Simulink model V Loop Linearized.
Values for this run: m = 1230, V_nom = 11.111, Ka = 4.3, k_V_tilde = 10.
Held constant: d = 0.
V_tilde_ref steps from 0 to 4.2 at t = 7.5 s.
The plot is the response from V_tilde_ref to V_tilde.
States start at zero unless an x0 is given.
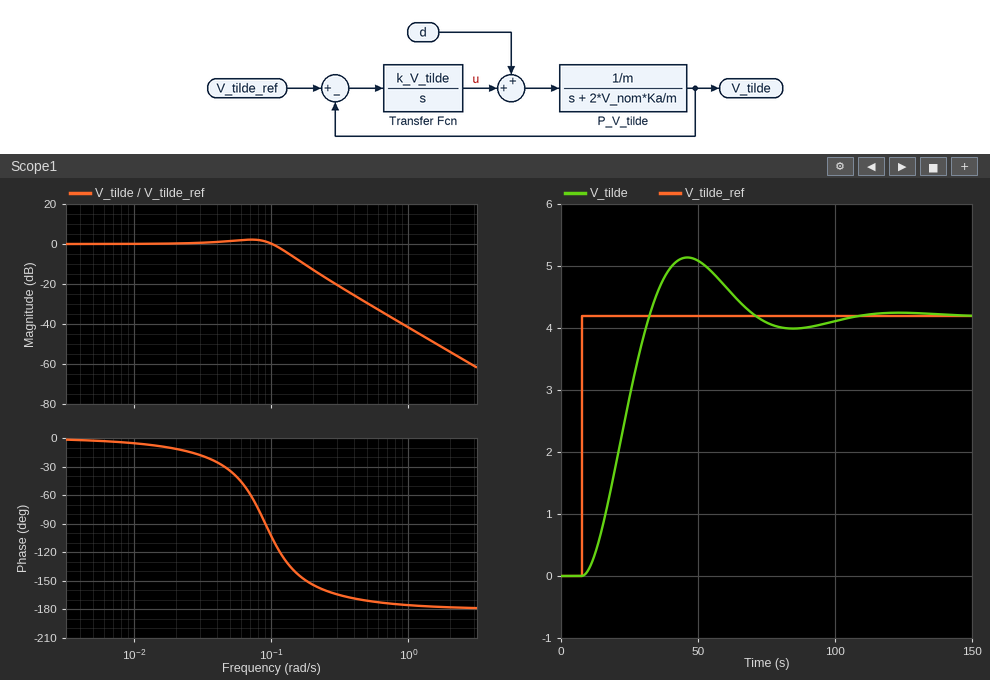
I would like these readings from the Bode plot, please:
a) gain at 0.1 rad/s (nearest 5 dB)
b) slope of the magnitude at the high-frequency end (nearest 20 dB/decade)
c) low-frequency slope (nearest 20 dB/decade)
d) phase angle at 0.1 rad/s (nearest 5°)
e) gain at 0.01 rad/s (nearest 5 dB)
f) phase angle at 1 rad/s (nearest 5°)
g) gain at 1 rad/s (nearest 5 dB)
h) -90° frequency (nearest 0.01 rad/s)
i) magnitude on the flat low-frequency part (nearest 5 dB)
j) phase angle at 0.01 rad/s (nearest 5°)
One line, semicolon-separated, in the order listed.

0 dB; -40 dB/decade; 0 dB/decade; -105°; 0 dB; -175°; -40 dB; 0.09 rad/s; 0 dB; -5°
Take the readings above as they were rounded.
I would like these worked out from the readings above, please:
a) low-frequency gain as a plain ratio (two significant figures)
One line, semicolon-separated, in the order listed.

1.0
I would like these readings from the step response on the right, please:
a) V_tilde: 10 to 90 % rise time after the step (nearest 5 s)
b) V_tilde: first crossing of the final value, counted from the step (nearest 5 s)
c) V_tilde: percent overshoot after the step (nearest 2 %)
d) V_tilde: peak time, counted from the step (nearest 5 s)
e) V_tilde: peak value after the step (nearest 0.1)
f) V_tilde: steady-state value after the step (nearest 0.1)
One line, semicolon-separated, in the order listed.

15 s; 25 s; 22 %; 40 s; 5.1; 4.2
